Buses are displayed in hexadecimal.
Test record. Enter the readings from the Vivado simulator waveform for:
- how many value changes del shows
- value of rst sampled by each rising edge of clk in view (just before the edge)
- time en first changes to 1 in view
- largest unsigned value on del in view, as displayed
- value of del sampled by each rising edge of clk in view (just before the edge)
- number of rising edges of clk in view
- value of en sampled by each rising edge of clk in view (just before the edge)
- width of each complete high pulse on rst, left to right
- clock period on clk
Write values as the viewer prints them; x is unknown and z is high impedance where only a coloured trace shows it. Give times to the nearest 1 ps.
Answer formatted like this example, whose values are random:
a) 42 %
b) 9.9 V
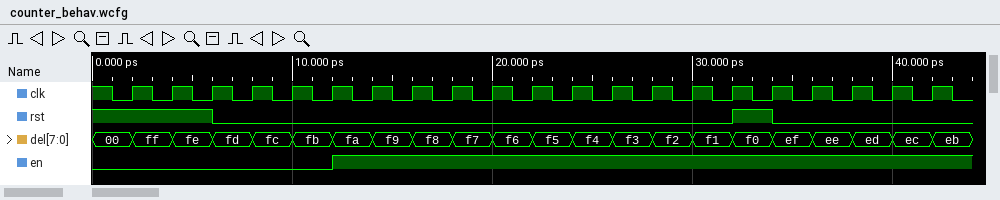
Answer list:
a) 21
b) 1 1 1 0 0 0 0 0 0 0 0 0 0 0 0 0 1 0 0 0 0
c) 12 ps
d) ff
e) 00, ff, fe, fd, fc, fb, fa, f9, f8, f7, f6, f5, f4, f3, f2, f1, f0, ef, ee, ed, ec
f) 21
g) 0 0 0 0 0 0 1 1 1 1 1 1 1 1 1 1 1 1 1 1 1
h) 2 ps
i) 2 ps
